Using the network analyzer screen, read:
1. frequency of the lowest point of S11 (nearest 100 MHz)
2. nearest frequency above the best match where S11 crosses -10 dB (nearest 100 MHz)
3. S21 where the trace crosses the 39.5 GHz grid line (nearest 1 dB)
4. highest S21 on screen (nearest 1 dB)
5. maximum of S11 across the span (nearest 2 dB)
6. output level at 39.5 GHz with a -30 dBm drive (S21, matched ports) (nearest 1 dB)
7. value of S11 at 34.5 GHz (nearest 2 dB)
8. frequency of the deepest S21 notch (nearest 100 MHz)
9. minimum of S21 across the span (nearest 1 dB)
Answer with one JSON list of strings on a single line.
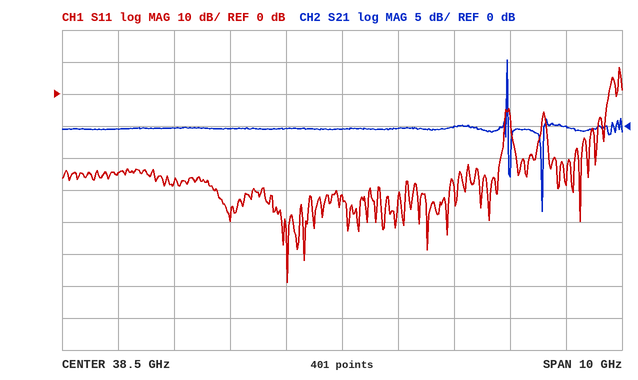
["37.5 GHz", "41.4 GHz", "0 dB", "10 dB", "8 dB", "-30 dBm", "-24 dB", "42.1 GHz", "-13 dB"]
